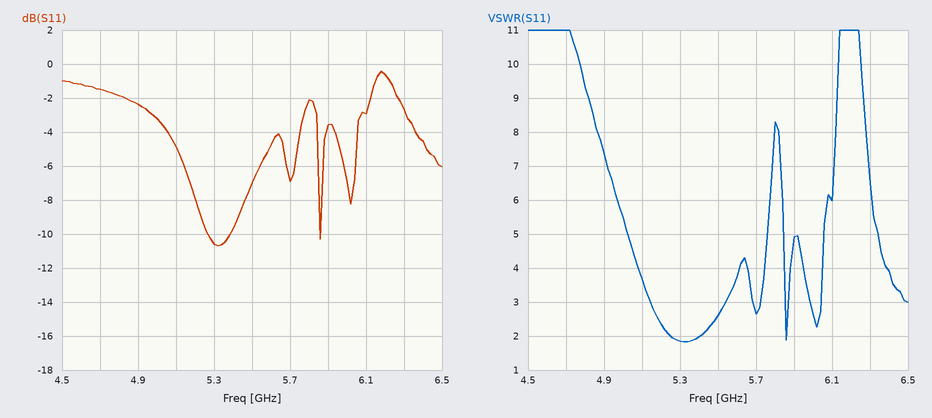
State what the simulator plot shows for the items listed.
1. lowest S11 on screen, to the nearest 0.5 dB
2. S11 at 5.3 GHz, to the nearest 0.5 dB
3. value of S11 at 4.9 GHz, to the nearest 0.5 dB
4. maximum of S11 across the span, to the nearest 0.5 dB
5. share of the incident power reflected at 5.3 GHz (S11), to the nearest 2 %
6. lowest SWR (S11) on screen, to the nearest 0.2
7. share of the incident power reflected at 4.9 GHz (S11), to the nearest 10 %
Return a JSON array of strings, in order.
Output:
["-10.5 dB", "-10.5 dB", "-2.5 dB", "-0.5 dB", "8 %", "1.8", "60 %"]
